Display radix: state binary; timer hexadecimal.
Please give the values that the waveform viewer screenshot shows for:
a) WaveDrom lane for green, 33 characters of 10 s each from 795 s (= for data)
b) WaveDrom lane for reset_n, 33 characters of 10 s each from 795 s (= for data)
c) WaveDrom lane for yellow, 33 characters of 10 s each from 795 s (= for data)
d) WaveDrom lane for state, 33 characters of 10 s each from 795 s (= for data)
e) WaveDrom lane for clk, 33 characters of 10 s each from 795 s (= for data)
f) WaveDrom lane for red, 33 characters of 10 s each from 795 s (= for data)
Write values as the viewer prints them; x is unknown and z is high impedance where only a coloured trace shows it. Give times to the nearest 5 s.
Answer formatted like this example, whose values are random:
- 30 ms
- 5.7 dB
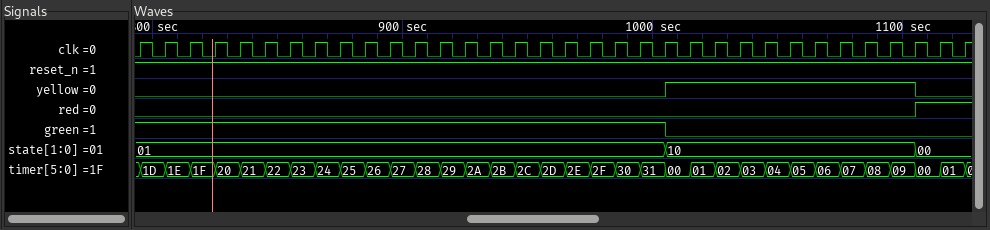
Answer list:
- {name: 'green', wave: '1....................0...........'}
- {name: 'reset_n', wave: '1................................'}
- {name: 'yellow', wave: '0....................1.........0.'}
- {name: 'state', wave: '=....................=.........=.', data: '01 10 00'}
- {name: 'clk', wave: 'p................................'}
- {name: 'red', wave: '0..............................1.'}
